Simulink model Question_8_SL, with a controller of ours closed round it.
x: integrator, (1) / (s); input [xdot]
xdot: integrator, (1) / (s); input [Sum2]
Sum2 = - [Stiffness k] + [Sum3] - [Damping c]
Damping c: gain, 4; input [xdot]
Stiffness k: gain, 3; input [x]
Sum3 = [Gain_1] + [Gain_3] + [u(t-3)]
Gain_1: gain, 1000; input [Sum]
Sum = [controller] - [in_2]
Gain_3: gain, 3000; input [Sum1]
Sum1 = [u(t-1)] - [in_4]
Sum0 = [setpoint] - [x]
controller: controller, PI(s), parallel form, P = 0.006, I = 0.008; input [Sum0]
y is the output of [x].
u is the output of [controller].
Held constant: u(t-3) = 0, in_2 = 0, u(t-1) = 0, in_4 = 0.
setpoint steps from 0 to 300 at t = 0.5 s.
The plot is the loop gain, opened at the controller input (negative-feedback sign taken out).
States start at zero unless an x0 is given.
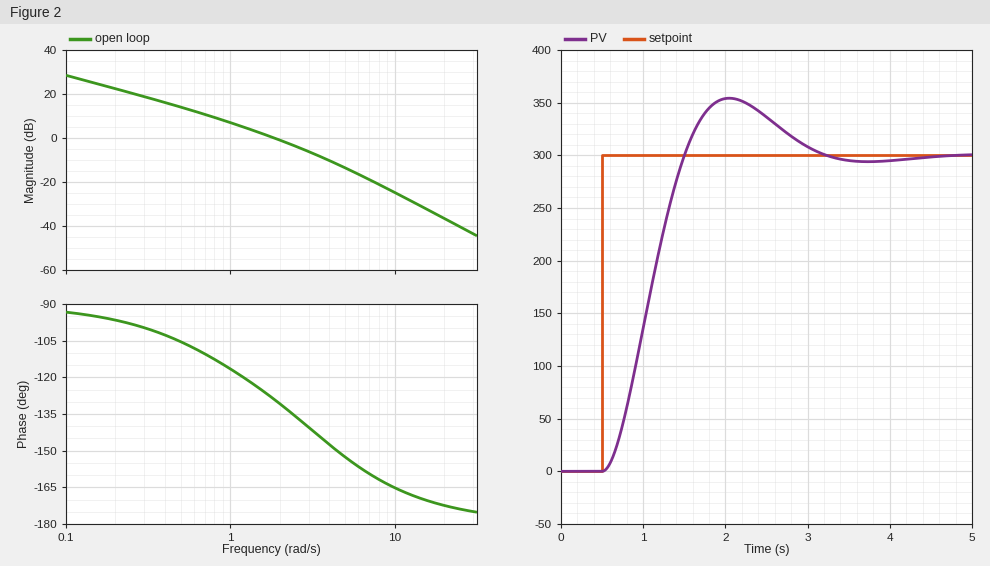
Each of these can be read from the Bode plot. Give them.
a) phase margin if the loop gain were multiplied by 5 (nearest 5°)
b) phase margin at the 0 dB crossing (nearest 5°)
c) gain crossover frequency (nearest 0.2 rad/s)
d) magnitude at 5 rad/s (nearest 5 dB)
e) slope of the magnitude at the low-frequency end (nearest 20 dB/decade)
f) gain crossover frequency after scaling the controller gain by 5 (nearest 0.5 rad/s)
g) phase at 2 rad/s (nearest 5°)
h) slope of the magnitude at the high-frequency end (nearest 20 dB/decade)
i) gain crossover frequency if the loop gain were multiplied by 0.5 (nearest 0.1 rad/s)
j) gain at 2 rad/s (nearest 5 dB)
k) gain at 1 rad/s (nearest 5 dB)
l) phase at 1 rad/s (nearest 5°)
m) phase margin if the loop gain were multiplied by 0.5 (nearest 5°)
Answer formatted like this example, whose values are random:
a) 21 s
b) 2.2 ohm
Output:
a) 25°
b) 50°
c) 1.8 rad/s
d) -15 dB
e) -20 dB/decade
f) 5.0 rad/s
g) -130°
h) -40 dB/decade
i) 1.1 rad/s
j) 0 dB
k) 5 dB
l) -115°
m) 60°
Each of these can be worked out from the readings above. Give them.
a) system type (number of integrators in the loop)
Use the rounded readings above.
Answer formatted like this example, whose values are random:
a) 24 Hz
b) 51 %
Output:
a) 1
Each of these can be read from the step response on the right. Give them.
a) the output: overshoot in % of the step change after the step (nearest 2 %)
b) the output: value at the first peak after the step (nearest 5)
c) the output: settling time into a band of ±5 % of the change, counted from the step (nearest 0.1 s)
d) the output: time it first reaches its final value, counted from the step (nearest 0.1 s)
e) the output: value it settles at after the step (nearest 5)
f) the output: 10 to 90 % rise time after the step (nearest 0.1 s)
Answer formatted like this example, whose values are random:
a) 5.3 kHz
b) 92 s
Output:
a) 18 %
b) 355
c) 2.4 s
d) 1.0 s
e) 300
f) 0.7 s
